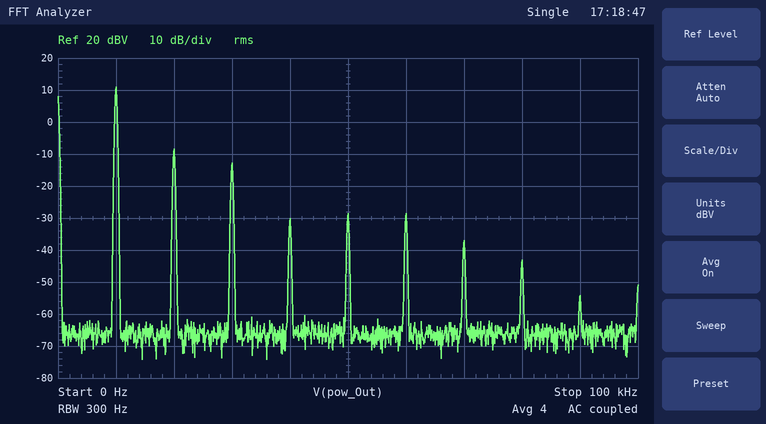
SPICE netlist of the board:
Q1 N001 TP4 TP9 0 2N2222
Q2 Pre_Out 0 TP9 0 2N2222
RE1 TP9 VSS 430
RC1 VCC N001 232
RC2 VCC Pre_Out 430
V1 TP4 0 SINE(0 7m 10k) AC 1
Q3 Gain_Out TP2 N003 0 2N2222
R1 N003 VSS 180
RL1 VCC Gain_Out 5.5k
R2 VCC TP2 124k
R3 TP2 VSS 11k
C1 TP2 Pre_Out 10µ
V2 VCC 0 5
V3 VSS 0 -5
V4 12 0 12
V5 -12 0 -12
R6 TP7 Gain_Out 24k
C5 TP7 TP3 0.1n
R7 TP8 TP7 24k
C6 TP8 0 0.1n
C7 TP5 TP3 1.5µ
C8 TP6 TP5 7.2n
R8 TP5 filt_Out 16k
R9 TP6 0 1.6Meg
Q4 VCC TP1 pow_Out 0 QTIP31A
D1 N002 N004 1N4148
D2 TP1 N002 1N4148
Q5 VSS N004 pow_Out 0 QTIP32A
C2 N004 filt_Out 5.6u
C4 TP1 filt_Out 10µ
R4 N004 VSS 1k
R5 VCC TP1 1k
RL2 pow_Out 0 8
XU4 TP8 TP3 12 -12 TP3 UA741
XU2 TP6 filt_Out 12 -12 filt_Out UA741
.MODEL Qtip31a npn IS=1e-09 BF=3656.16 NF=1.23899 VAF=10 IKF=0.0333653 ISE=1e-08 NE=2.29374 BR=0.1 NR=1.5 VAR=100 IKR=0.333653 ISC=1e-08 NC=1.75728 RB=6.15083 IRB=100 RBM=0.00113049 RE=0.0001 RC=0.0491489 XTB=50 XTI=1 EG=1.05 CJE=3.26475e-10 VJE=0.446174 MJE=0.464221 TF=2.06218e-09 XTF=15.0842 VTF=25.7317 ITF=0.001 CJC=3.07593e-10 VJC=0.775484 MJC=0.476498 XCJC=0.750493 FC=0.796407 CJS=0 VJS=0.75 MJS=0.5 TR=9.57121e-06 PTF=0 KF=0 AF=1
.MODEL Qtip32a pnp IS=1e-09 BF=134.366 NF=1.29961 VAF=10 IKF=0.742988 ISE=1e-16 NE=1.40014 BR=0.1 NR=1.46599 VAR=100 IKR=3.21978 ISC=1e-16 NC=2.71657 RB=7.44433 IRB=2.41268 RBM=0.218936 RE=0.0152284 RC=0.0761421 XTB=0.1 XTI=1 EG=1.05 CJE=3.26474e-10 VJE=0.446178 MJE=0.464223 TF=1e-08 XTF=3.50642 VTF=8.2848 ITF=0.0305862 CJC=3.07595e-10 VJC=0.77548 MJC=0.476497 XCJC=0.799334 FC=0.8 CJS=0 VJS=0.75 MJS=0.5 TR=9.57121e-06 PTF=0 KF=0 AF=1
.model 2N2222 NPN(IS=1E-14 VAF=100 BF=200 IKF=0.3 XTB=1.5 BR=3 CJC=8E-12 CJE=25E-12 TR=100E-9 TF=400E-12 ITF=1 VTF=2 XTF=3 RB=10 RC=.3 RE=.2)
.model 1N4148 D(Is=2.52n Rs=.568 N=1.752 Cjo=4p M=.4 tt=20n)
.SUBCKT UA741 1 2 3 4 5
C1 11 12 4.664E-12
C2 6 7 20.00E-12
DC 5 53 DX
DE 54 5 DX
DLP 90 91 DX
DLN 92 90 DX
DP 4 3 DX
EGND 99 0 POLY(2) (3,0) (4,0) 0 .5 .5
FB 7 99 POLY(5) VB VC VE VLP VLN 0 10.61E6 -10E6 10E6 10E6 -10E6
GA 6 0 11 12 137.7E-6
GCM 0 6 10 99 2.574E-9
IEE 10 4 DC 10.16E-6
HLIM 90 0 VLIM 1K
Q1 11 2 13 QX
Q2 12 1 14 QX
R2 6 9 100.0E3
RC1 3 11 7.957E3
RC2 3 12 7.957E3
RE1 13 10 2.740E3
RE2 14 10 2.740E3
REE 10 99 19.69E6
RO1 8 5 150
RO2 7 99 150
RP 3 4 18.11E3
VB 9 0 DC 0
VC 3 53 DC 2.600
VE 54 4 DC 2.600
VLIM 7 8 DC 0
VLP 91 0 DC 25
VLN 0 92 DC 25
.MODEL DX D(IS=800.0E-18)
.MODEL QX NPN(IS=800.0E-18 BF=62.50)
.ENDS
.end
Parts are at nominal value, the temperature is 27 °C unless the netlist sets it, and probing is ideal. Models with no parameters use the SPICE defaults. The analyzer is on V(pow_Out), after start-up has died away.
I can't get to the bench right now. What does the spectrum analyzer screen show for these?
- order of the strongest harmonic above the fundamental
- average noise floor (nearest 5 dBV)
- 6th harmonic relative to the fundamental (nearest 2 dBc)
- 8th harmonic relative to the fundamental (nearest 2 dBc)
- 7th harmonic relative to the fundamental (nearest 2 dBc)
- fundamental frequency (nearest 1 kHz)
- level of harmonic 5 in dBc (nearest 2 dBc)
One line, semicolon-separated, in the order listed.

2; -65 dBV; -40 dBc; -54 dBc; -48 dBc; 10 kHz; -40 dBc
